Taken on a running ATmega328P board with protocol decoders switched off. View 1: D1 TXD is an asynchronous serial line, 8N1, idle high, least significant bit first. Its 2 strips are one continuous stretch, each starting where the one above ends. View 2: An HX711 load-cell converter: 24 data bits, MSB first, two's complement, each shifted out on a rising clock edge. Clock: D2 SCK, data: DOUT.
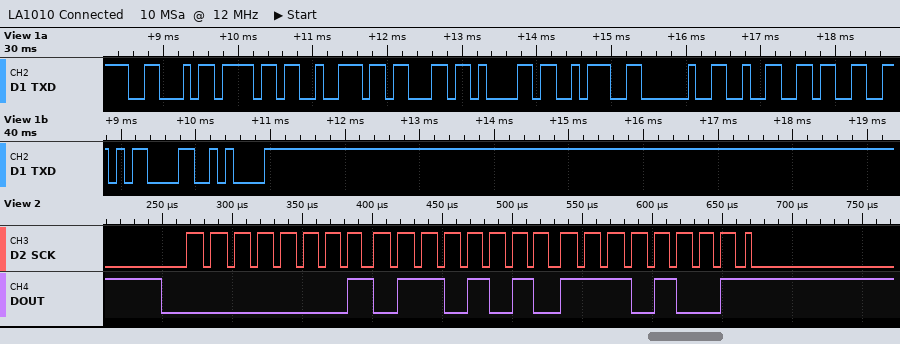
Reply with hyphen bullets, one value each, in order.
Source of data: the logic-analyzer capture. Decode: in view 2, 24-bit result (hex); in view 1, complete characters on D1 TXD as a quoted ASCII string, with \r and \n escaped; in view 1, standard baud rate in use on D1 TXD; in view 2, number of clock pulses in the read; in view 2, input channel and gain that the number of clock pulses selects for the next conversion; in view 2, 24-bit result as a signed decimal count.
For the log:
- 0x016AE9
- "Forca: 23\r\n"
- 9600 baud
- 25
- channel A, gain 128
- 92905
